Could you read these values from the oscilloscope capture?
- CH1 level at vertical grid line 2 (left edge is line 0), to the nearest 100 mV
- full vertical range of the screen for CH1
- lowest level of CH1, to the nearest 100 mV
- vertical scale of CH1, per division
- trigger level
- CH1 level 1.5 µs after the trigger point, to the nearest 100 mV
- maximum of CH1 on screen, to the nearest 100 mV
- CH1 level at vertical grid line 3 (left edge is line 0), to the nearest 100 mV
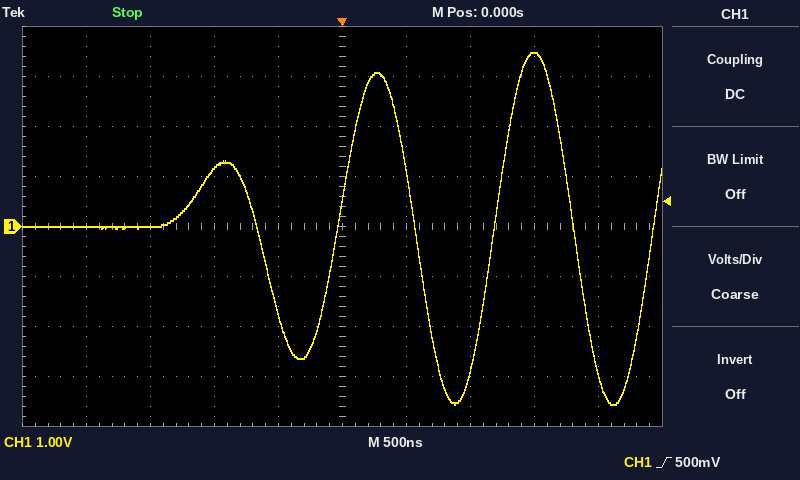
0.0 V
8 V
-3.6 V
1 V
500 mV
3.5 V
3.5 V
1.2 V
